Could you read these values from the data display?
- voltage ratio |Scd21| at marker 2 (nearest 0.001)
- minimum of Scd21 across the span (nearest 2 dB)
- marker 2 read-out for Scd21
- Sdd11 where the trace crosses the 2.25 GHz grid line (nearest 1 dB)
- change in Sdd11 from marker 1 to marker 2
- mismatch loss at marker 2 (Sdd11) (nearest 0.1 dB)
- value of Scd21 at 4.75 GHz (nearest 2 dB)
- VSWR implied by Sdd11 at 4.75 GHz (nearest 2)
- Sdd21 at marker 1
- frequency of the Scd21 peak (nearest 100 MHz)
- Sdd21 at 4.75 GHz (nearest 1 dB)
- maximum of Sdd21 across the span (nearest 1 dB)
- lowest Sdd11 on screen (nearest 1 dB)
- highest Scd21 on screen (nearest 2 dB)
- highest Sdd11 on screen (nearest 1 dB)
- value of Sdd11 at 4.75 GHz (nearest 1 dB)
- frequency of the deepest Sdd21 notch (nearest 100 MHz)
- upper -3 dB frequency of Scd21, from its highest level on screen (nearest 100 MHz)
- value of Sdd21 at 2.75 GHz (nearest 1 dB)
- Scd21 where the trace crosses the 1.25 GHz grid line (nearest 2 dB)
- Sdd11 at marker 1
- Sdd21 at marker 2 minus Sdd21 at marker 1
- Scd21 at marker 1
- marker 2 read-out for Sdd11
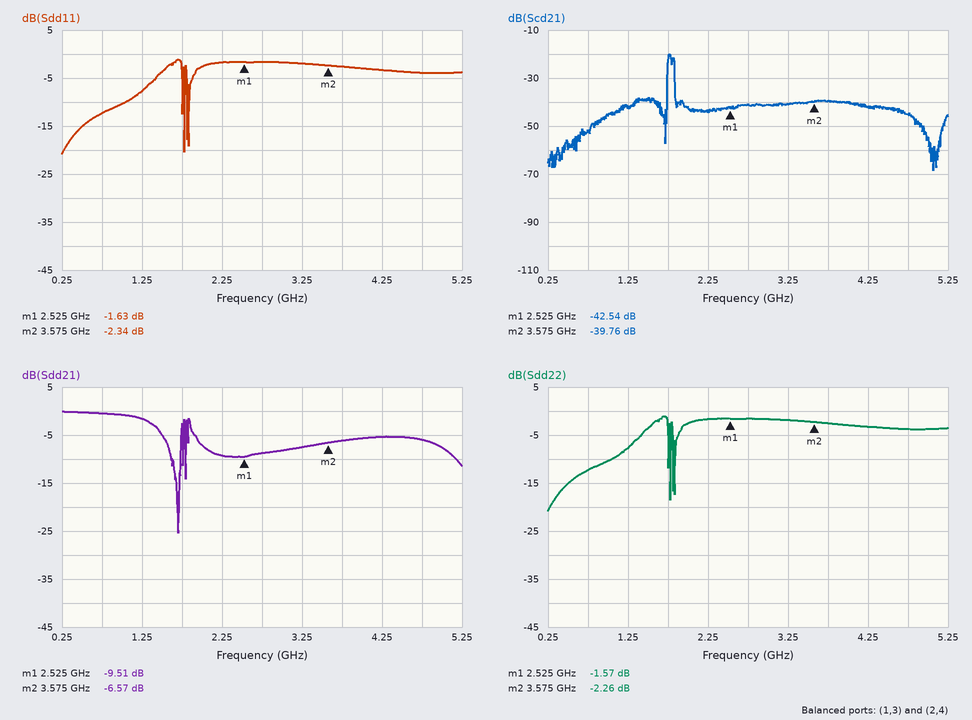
0.010
-68 dB
-39.76 dB
-2 dB
-0.71 dB
3.8 dB
-46 dB
4
-9.51 dB
1.8 GHz
-6 dB
0 dB
-21 dB
-20 dB
-1 dB
-4 dB
1.7 GHz
1.8 GHz
-9 dB
-42 dB
-1.63 dB
2.94 dB
-42.54 dB
-2.34 dB
